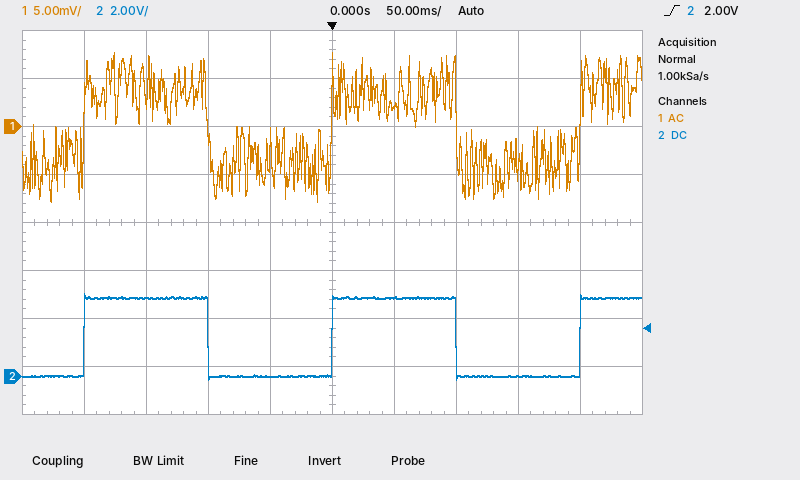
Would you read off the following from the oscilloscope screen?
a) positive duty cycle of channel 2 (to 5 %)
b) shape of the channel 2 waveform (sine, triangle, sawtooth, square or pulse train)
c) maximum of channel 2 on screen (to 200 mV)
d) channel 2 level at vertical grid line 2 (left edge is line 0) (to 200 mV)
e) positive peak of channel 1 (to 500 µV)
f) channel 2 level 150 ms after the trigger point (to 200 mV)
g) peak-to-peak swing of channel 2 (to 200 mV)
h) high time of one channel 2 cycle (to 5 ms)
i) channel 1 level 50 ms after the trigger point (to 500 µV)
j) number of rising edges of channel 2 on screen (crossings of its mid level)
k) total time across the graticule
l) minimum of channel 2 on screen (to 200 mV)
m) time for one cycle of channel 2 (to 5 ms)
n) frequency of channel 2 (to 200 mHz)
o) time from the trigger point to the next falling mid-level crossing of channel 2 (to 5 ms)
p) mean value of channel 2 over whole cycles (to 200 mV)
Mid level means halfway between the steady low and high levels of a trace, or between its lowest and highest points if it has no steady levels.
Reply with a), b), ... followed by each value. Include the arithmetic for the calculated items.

a) 100 ms / 200 ms ≈ 50 %
b) square
c) 3.4 V
d) 3.2 V
e) 7.5 mV
f) 0.0 V
g) 3.4 V − (-200 mV) = 3.6 V
h) 100 ms
i) 2.0 mV
j) 3
k) 500 ms
l) -200 mV
m) 200 ms
n) 1 / 200 ms ≈ 5.0 Hz
o) 100 ms
p) -200 mV + 0.5 × (3.4 V − (-200 mV)) ≈ 1.6 V
